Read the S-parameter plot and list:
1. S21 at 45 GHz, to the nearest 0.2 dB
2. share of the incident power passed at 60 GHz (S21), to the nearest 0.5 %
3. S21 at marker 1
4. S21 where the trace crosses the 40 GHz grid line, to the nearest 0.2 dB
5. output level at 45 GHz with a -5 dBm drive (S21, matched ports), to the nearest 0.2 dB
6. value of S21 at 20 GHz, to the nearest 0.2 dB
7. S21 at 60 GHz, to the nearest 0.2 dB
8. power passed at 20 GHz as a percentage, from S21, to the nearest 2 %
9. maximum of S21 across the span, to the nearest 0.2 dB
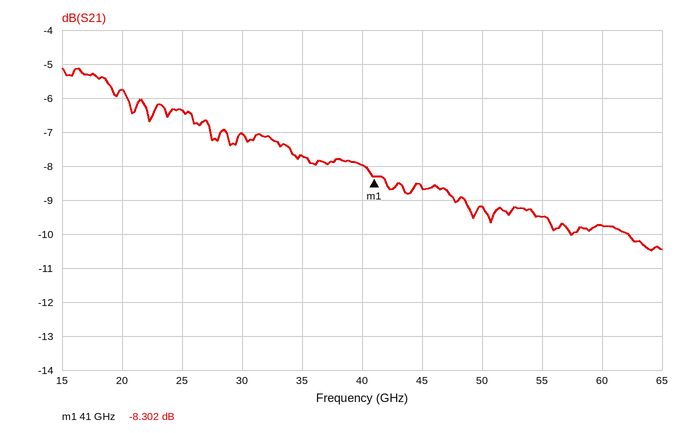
-8.6 dB
10.5 %
-8.302 dB
-8.0 dB
-13.6 dBm
-5.8 dB
-9.8 dB
26 %
-5.2 dB
